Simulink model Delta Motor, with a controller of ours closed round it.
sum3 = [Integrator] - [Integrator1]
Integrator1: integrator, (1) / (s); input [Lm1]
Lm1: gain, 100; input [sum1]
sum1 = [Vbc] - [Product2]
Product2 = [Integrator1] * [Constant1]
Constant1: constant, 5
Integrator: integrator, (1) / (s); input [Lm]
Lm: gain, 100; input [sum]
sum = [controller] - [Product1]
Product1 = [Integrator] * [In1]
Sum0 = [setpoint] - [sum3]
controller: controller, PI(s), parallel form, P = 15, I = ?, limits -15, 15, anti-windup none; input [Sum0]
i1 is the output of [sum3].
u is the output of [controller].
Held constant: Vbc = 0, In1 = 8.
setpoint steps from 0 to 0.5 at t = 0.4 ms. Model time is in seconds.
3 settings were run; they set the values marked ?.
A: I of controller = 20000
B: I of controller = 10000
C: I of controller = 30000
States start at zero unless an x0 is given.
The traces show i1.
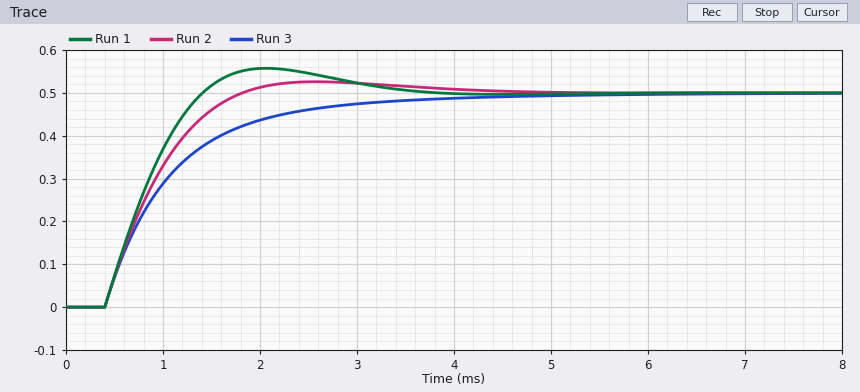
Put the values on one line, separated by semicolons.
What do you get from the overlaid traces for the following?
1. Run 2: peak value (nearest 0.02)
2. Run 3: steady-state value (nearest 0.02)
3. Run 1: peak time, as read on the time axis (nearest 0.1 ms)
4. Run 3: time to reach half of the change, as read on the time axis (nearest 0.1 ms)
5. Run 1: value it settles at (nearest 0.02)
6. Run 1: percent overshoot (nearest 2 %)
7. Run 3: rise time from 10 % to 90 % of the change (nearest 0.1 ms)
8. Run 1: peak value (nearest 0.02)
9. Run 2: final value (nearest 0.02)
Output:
0.52; 0.50; 2.1 ms; 0.9 ms; 0.50; 12 %; 1.8 ms; 0.56; 0.50
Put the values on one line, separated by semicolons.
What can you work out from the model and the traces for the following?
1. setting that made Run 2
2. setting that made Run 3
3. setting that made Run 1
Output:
A; B; C
